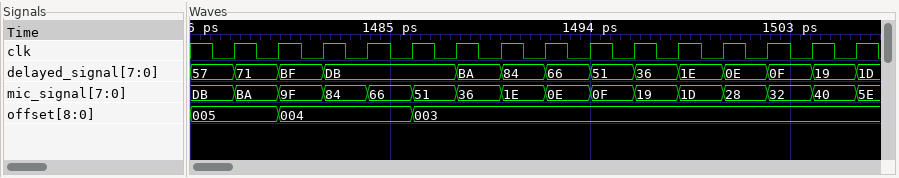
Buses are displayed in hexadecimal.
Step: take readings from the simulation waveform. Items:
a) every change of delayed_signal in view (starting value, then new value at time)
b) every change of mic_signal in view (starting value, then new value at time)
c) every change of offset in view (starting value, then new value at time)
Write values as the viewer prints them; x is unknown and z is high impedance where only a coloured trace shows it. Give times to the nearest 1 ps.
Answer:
57, 71 at 1478 ps, BF at 1480 ps, DB at 1482 ps, BA at 1488 ps, 84 at 1490 ps, 66 at 1492 ps, 51 at 1494 ps, 36 at 1496 ps, 1E at 1498 ps, 0E at 1500 ps, 0F at 1502 ps, 19 at 1504 ps, 1D at 1506 ps
DB, BA at 1478 ps, 9F at 1480 ps, 84 at 1482 ps, 66 at 1484 ps, 51 at 1486 ps, 36 at 1488 ps, 1E at 1490 ps, 0E at 1492 ps, 0F at 1494 ps, 19 at 1496 ps, 1D at 1498 ps, 28 at 1500 ps, 32 at 1502 ps, 40 at 1504 ps, 5E at 1506 ps
005, 004 at 1480 ps, 003 at 1486 ps
